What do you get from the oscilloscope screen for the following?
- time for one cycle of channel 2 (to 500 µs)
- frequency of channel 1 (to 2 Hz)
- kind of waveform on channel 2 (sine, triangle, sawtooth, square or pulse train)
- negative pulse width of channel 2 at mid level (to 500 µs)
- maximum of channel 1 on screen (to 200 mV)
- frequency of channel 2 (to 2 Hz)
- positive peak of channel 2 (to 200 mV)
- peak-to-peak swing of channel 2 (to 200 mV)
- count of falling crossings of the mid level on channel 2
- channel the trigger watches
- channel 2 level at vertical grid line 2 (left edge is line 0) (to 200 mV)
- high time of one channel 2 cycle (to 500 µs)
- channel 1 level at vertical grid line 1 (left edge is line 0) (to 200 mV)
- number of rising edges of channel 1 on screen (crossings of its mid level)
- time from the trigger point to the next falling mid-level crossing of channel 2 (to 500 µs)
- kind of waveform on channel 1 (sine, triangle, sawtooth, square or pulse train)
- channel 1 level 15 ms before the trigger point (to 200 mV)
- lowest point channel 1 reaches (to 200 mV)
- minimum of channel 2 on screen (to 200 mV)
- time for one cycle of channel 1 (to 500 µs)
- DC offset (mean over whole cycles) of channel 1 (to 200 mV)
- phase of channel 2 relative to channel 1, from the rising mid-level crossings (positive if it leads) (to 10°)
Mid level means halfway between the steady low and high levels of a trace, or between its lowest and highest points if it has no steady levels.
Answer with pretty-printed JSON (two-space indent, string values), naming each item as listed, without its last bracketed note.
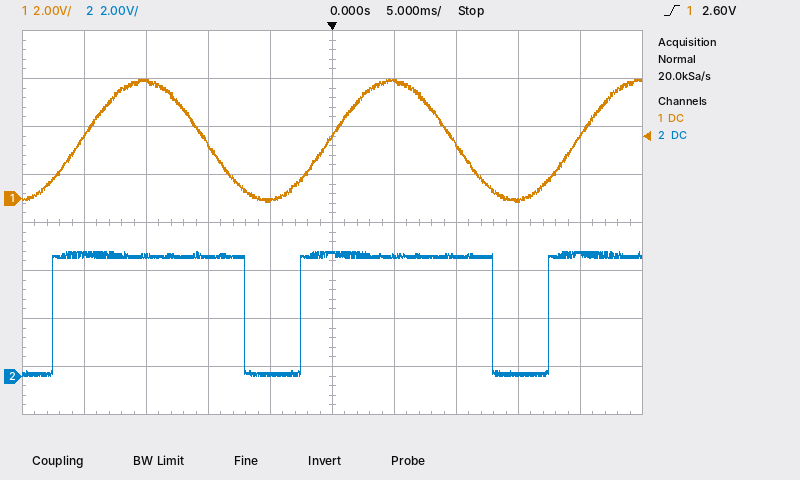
{
  "time for one cycle of channel 2": "20.0 ms",
  "frequency of channel 1": "50 Hz",
  "kind of waveform on channel 2": "pulse train",
  "negative pulse width of channel 2 at mid level": "4.5 ms",
  "maximum of channel 1 on screen": "5.0 V",
  "frequency of channel 2": "50 Hz",
  "positive peak of channel 2": "5.2 V",
  "peak-to-peak swing of channel 2": "5.2 V",
  "count of falling crossings of the mid level on channel 2": "2",
  "channel the trigger watches": "channel 1",
  "channel 2 level at vertical grid line 2 (left edge is line 0)": "5.0 V",
  "high time of one channel 2 cycle": "15.5 ms",
  "channel 1 level at vertical grid line 1 (left edge is line 0)": "2.6 V",
  "number of rising edges of channel 1 on screen": "3",
  "time from the trigger point to the next falling mid-level crossing of channel 2": "13.0 ms",
  "kind of waveform on channel 1": "sine",
  "channel 1 level 15 ms before the trigger point": "4.8 V",
  "lowest point channel 1 reaches": "-200 mV",
  "minimum of channel 2 on screen": "0.0 V",
  "time for one cycle of channel 1": "20.0 ms",
  "DC offset (mean over whole cycles) of channel 1": "2.4 V",
  "phase of channel 2 relative to channel 1, from the rising mid-level crossings (positive if it leads)": "+40°"
}
